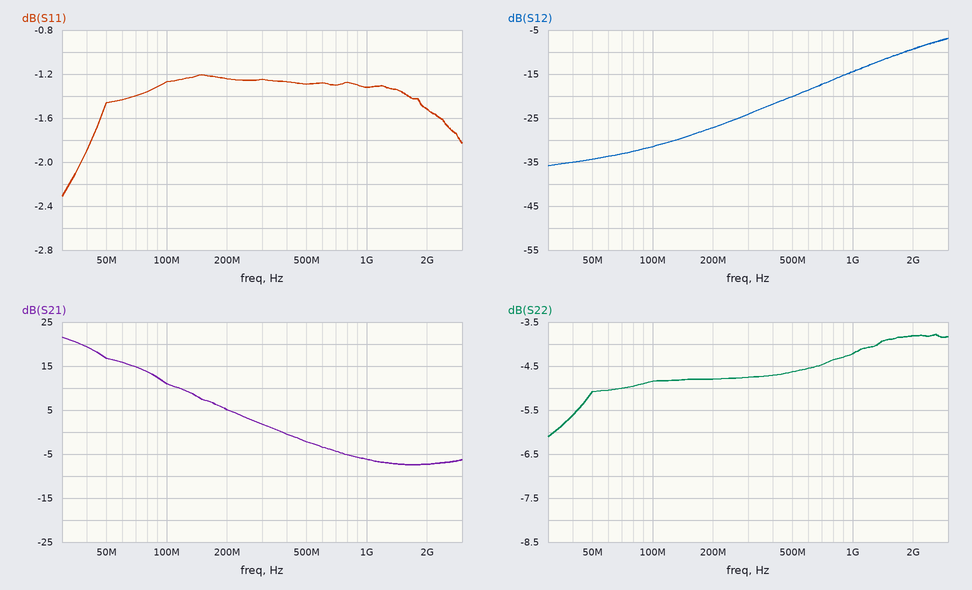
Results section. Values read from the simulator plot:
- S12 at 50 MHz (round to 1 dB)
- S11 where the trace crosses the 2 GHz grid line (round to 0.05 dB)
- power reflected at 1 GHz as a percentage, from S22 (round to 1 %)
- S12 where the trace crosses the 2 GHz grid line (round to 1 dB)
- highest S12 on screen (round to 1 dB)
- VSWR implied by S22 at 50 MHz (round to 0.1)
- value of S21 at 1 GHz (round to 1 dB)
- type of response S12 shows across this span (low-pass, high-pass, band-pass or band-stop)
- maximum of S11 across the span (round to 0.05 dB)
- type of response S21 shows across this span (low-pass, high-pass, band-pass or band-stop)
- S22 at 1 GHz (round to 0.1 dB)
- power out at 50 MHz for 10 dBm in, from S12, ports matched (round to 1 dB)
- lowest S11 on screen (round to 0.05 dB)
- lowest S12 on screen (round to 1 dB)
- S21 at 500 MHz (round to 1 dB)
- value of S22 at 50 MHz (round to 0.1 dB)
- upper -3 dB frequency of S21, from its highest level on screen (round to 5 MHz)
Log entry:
-34 dB
-1.50 dB
38 %
-9 dB
-7 dB
3.5
-6 dB
high-pass
-1.20 dB
low-pass
-4.2 dB
-24 dBm
-2.30 dB
-36 dB
-2 dB
-5.1 dB
45 MHz
